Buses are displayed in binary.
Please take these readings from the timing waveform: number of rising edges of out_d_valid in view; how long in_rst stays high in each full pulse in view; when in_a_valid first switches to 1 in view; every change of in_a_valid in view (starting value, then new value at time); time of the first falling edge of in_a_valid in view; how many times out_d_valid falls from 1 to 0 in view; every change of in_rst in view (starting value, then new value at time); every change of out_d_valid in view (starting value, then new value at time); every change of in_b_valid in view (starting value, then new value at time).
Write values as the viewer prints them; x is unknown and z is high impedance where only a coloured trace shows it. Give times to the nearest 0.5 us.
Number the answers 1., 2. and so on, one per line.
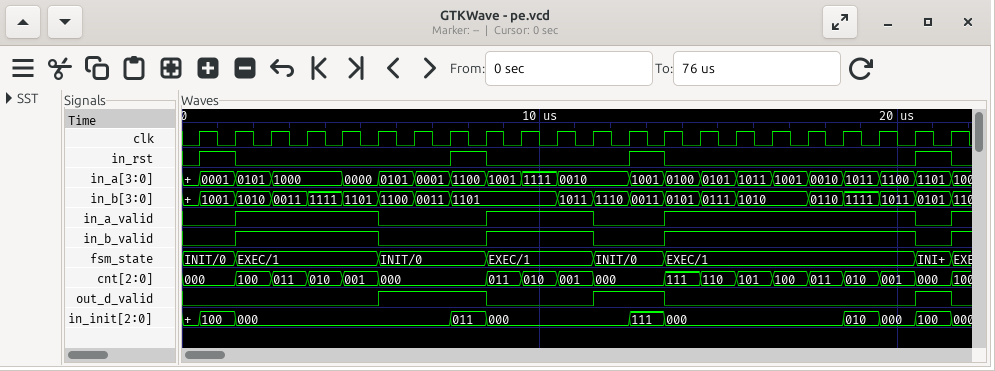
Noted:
1. 3
2. 1 us, 1 us, 1 us, 1 us
3. 1.5 us
4. 0, 1 at 1.5 us, 0 at 5.5 us, 1 at 8.5 us, 0 at 11.5 us, 1 at 13.5 us, 0 at 20.5 us, 1 at 21.5 us
5. 5.5 us
6. 3
7. 0, 1 at 0.5 us, 0 at 1.5 us, 1 at 7.5 us, 0 at 8.5 us, 1 at 12.5 us, 0 at 13.5 us, 1 at 20.5 us, 0 at 21.5 us
8. 0, 1 at 5.5 us, 0 at 8.5 us, 1 at 11.5 us, 0 at 13.5 us, 1 at 20.5 us, 0 at 21.5 us
9. 0, 1 at 1.5 us, 0 at 5.5 us, 1 at 8.5 us, 0 at 11.5 us, 1 at 13.5 us, 0 at 20.5 us, 1 at 21.5 us
